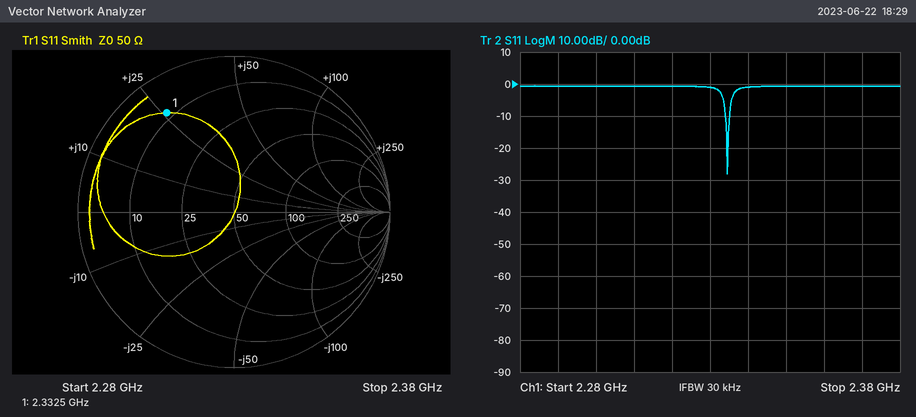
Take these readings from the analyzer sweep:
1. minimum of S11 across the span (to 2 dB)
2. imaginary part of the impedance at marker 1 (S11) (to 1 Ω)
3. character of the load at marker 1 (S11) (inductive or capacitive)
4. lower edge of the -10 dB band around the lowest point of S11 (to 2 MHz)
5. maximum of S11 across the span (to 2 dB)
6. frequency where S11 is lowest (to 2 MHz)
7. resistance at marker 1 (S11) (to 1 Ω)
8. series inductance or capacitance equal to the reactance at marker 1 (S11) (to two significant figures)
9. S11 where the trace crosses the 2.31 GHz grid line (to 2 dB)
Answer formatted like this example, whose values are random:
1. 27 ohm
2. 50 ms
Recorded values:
1. -28 dB
2. +26 Ω
3. inductive
4. 2.334 GHz
5. 0 dB
6. 2.334 GHz
7. 8 Ω
8. 1.8 nH
9. 0 dB
